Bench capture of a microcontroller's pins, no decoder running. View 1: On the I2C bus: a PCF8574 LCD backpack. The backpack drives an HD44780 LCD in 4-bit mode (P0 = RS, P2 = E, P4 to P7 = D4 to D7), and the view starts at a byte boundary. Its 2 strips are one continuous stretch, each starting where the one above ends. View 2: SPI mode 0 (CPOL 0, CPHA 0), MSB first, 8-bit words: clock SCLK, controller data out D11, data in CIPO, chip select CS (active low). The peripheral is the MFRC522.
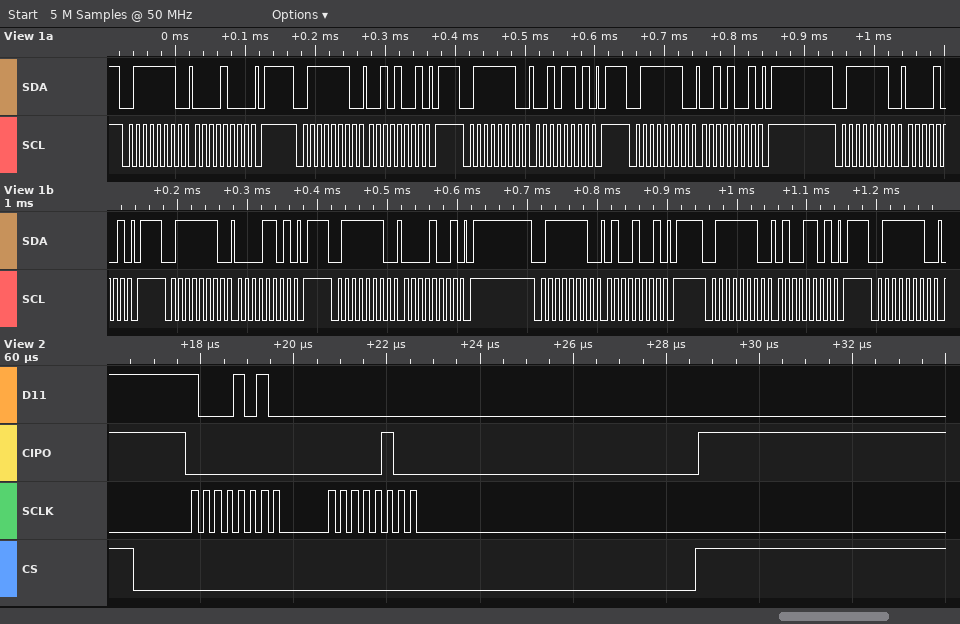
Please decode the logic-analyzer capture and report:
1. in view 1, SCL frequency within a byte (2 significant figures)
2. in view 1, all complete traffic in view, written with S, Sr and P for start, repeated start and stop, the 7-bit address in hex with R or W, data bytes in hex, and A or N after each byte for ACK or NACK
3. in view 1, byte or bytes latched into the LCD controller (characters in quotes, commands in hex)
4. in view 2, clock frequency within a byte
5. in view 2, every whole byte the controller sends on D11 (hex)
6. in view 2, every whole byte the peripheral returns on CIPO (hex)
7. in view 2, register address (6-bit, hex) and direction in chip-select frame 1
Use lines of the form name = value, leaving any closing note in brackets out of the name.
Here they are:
in view 1, SCL frequency within a byte = 100 kHz
in view 1, all complete traffic in view, written with S, Sr and P for start, repeated start and stop, the 7-bit address in hex with R or W, data bytes in hex, and A or N after each byte for ACK or NACK = S 3FW A 08 A P S 3FW A 29 A P S 3FW A 2D A P S 3FW A 29 A P S 3FW A 09 A P S 3FW A 0D A P S 3FW A 09 A P S 3FW A 49 A P S 3FW A 4D A P S 3FW A
in view 1, byte or bytes latched into the LCD controller = ' '
in view 2, clock frequency within a byte = 4 MHz
in view 2, every whole byte the controller sends on D11 = 0x8A 0x00
in view 2, every whole byte the peripheral returns on CIPO = 0x00 0x04
in view 2, register address (6-bit, hex) and direction in chip-select frame 1 = 0x05 read
